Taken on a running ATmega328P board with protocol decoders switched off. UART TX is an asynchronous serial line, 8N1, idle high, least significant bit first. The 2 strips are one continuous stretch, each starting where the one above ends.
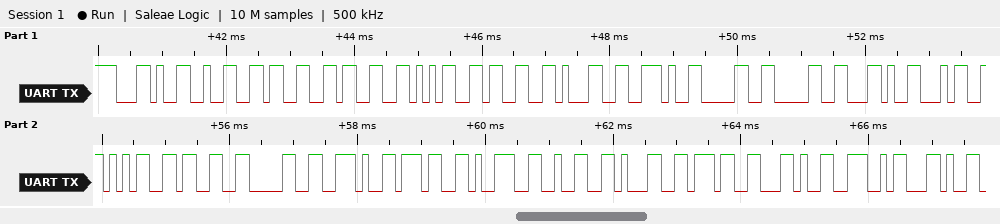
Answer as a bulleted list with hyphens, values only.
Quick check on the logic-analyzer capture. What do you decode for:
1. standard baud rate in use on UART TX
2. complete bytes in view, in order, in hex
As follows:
- 9600 baud
- 2C 32 33 33 35 33 31 2E 30 30 2C 34 35 33 30 2E 37 39 32 31 37 2C 4E 2C
